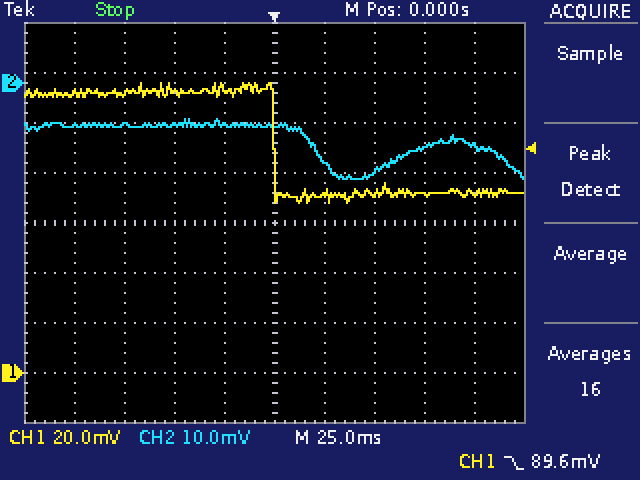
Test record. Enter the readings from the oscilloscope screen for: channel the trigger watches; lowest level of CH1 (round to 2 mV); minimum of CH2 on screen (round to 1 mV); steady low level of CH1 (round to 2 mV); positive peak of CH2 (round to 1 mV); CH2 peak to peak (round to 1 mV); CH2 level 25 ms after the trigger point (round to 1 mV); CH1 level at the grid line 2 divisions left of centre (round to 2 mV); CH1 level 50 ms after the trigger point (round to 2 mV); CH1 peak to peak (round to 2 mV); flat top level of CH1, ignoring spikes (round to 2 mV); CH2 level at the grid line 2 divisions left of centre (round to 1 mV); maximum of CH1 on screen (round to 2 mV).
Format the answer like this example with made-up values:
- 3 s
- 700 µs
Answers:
- CH1
- 68 mV
- -19 mV
- 72 mV
- -7 mV
- 12 mV
- -16 mV
- 112 mV
- 72 mV
- 48 mV
- 112 mV
- -8 mV
- 116 mV
